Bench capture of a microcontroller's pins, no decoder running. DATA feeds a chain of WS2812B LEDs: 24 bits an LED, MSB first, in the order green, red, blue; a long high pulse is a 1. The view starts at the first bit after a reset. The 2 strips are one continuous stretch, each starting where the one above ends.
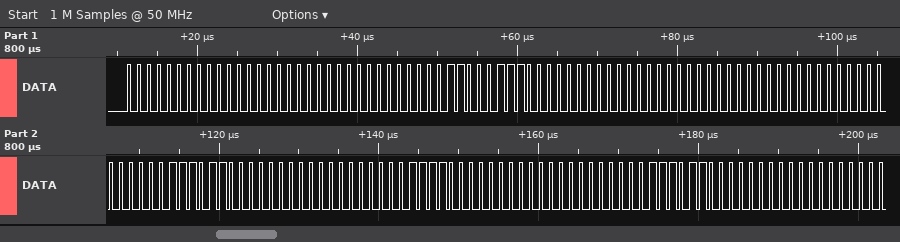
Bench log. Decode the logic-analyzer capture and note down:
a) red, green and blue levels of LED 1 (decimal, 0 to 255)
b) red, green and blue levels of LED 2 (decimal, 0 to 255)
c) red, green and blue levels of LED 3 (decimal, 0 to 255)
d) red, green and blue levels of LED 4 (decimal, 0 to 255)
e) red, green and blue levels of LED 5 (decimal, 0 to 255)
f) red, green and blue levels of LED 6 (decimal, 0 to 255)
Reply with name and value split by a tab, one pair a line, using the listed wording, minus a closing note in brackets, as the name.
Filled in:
red, green and blue levels of LED 1	0, 0, 0
red, green and blue levels of LED 2	199, 0, 0
red, green and blue levels of LED 3	0, 0, 0
red, green and blue levels of LED 4	59, 0, 0
red, green and blue levels of LED 5	60, 0, 0
red, green and blue levels of LED 6	59, 0, 0
